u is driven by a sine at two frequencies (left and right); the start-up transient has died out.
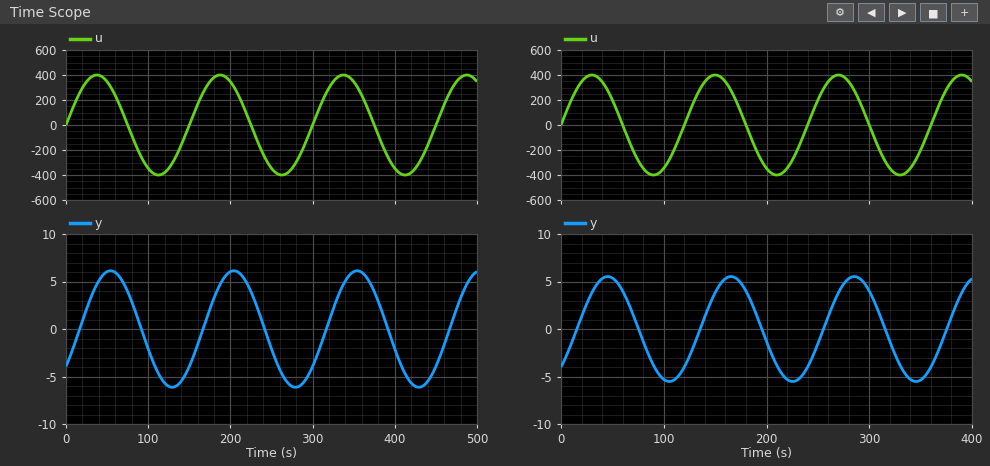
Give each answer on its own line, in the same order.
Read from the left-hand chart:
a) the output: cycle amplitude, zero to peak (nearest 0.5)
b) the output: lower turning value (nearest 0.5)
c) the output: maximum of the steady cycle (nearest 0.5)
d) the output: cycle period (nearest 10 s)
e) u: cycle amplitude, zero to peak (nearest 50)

6.0
-6.0
6.0
150 s
400
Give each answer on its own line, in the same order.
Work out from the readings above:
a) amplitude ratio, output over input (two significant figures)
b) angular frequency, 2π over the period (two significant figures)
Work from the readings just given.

0.015
0.042 rad/s
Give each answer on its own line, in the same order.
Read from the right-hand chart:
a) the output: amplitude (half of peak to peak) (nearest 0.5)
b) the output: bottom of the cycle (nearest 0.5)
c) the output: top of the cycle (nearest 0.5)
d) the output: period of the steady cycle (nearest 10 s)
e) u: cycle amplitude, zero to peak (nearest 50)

5.5
-5.5
5.5
120 s
400
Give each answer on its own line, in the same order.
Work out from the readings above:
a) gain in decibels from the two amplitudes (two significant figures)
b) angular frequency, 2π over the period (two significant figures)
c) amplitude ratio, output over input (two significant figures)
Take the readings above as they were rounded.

-37 dB
0.052 rad/s
0.014
